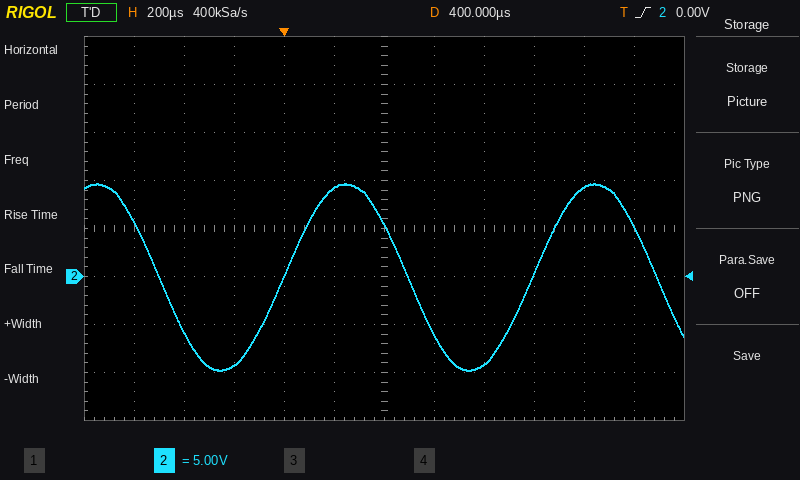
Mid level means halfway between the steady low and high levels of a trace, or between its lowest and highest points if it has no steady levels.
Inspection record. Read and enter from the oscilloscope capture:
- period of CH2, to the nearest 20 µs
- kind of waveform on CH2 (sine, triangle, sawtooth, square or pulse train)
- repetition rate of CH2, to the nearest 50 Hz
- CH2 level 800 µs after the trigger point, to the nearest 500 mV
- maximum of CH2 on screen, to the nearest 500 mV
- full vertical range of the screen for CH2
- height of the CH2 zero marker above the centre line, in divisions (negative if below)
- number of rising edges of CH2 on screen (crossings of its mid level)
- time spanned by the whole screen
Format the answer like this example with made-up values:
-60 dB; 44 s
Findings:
1.00 ms; sine; 1.00 kHz; -9.0 V; 9.5 V; 40 V; -1.0 div; 2; 2.4 ms
